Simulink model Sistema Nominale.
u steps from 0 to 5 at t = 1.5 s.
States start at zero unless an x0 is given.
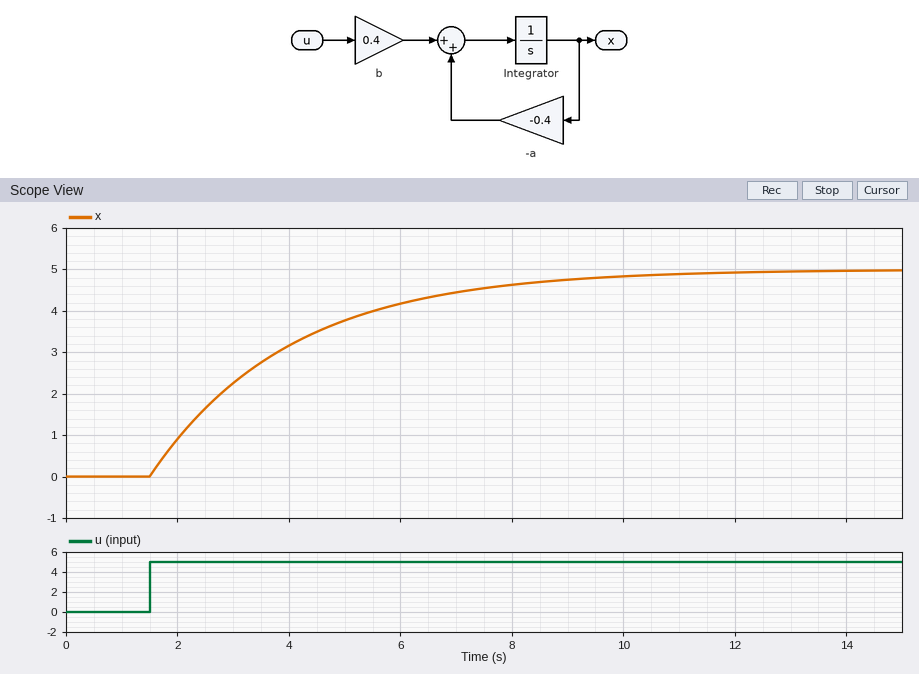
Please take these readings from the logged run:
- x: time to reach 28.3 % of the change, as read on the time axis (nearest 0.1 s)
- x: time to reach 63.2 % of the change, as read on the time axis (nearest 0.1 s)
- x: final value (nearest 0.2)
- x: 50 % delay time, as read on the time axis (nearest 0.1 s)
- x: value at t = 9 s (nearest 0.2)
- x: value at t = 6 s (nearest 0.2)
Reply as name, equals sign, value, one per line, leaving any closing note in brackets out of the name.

x: time to reach 28.3 % of the change, as read on the time axis = 2.3 s
x: time to reach 63.2 % of the change, as read on the time axis = 4.0 s
x: final value = 5.0
x: 50 % delay time, as read on the time axis = 3.2 s
x: value at t = 9 s = 4.8
x: value at t = 6 s = 4.2
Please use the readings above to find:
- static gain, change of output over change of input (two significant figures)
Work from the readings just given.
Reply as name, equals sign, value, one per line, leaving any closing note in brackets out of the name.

static gain, change of output over change of input = 1.0
